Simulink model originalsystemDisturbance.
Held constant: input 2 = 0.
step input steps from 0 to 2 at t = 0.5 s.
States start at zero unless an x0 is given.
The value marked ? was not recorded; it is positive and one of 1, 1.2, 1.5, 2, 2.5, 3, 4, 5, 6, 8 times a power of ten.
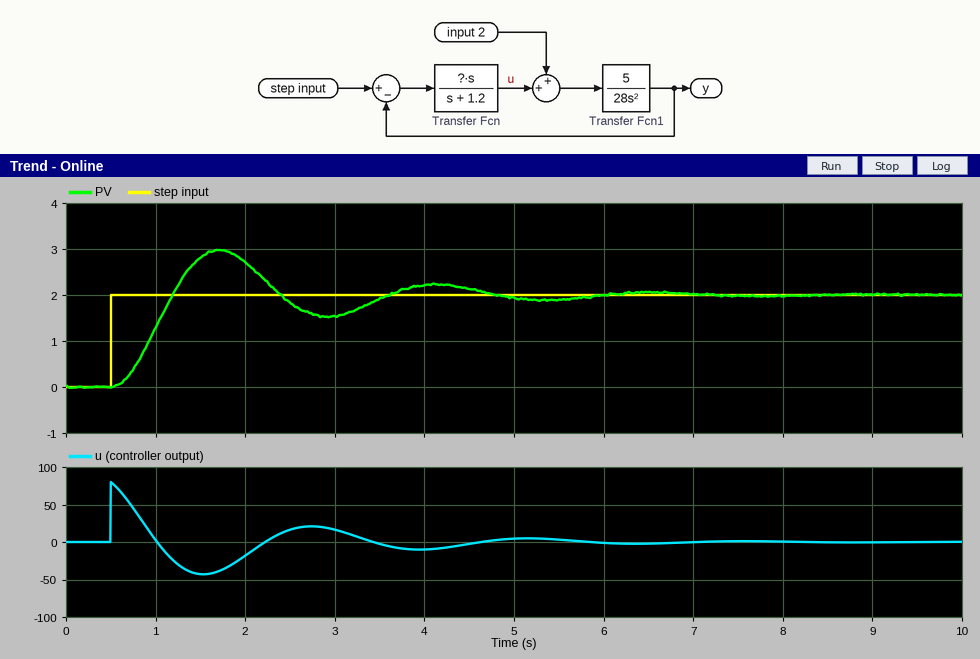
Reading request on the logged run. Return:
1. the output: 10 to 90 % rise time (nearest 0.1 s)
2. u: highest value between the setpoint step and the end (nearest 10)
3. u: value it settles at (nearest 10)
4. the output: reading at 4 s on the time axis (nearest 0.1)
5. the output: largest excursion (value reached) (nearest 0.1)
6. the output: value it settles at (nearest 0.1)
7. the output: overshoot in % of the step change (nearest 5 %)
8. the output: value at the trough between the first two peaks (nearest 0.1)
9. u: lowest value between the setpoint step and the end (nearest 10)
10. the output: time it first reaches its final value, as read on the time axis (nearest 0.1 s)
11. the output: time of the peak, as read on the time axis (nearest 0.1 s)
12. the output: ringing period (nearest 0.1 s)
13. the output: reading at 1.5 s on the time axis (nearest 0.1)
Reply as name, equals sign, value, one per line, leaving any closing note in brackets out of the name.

the output: 10 to 90 % rise time = 0.5 s
u: highest value between the setpoint step and the end = 80
u: value it settles at = 0
the output: reading at 4 s on the time axis = 2.2
the output: largest excursion (value reached) = 3.0
the output: value it settles at = 2.0
the output: overshoot in % of the step change = 50 %
the output: value at the trough between the first two peaks = 1.5
u: lowest value between the setpoint step and the end = -40
the output: time it first reaches its final value, as read on the time axis = 1.2 s
the output: time of the peak, as read on the time axis = 1.7 s
the output: ringing period = 2.4 s
the output: reading at 1.5 s on the time axis = 2.8
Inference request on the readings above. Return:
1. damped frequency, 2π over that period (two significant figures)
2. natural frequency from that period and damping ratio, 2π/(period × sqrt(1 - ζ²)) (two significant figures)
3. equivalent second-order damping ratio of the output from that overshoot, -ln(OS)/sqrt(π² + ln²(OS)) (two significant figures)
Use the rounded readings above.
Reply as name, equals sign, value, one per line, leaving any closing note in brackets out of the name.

damped frequency, 2π over that period = 2.6 rad/s
natural frequency from that period and damping ratio, 2π/(period × sqrt(1 - ζ²)) = 2.7 rad/s
equivalent second-order damping ratio of the output from that overshoot, -ln(OS)/sqrt(π² + ln²(OS)) = 0.22
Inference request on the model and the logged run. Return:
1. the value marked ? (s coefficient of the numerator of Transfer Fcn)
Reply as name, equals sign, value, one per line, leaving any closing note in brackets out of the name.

the value marked ? = 40
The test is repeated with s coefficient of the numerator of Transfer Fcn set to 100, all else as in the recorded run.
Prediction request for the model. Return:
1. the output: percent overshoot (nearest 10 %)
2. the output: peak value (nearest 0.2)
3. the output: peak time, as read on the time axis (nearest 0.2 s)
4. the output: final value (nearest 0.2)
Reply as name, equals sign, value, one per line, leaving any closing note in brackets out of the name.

the output: percent overshoot = 60 %
the output: peak value = 3.2
the output: peak time, as read on the time axis = 1.2 s
the output: final value = 2.0
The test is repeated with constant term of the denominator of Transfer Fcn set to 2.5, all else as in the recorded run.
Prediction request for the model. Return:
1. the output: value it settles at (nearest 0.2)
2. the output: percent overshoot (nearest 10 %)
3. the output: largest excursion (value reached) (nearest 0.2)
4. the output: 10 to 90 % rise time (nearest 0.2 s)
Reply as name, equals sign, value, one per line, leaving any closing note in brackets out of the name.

the output: value it settles at = 2.0
the output: percent overshoot = 20 %
the output: largest excursion (value reached) = 2.4
the output: 10 to 90 % rise time = 0.6 s
